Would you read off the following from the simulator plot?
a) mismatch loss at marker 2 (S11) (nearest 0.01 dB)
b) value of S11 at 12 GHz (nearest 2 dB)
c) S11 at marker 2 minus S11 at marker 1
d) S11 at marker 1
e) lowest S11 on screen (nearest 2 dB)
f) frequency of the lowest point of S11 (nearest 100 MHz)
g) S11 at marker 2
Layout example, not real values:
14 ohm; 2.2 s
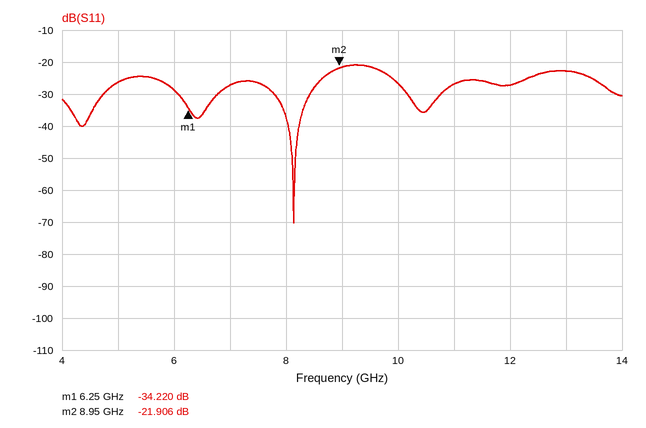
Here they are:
0.03 dB; -28 dB; 12.314 dB; -34.220 dB; -70 dB; 8.1 GHz; -21.906 dB
